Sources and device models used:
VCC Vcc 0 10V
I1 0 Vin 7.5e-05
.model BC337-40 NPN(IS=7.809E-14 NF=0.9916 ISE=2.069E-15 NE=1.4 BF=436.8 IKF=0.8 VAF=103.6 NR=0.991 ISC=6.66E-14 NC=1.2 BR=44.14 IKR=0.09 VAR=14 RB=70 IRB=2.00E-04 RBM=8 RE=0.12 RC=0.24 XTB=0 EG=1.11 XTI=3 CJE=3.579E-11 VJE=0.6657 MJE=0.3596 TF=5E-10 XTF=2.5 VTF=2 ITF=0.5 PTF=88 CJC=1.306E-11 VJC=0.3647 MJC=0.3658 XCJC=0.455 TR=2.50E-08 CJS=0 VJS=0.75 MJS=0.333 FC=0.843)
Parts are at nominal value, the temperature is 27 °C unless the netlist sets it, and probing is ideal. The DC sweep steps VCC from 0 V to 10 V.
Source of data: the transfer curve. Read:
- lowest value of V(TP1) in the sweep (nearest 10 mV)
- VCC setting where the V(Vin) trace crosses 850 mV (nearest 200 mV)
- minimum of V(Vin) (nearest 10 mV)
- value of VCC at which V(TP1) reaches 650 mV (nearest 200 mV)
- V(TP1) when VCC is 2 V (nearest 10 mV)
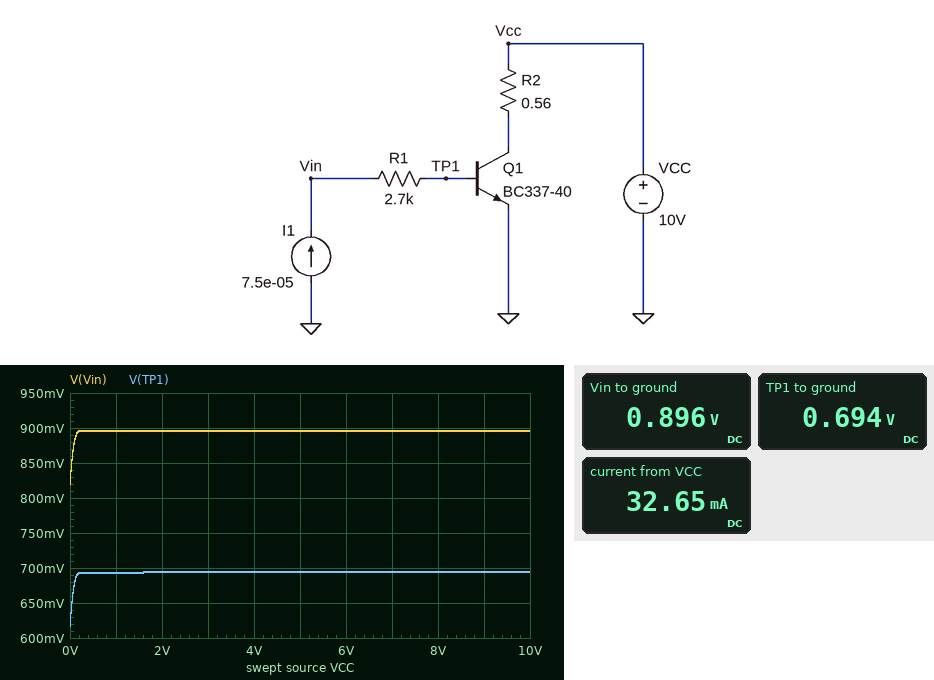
620 mV
0 V
820 mV
0 V
690 mV
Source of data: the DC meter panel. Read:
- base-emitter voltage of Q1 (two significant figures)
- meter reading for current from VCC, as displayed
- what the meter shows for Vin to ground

690 mV
32.65 mA
0.896 V
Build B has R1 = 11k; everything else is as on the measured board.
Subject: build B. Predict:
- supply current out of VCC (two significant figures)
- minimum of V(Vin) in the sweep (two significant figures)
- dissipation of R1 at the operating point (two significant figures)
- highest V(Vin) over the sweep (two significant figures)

33 mA
1.4 V
62 µW
1.5 V
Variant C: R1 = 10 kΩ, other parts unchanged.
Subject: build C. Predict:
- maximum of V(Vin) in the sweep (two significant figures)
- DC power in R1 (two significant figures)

1.4 V
56 µW
